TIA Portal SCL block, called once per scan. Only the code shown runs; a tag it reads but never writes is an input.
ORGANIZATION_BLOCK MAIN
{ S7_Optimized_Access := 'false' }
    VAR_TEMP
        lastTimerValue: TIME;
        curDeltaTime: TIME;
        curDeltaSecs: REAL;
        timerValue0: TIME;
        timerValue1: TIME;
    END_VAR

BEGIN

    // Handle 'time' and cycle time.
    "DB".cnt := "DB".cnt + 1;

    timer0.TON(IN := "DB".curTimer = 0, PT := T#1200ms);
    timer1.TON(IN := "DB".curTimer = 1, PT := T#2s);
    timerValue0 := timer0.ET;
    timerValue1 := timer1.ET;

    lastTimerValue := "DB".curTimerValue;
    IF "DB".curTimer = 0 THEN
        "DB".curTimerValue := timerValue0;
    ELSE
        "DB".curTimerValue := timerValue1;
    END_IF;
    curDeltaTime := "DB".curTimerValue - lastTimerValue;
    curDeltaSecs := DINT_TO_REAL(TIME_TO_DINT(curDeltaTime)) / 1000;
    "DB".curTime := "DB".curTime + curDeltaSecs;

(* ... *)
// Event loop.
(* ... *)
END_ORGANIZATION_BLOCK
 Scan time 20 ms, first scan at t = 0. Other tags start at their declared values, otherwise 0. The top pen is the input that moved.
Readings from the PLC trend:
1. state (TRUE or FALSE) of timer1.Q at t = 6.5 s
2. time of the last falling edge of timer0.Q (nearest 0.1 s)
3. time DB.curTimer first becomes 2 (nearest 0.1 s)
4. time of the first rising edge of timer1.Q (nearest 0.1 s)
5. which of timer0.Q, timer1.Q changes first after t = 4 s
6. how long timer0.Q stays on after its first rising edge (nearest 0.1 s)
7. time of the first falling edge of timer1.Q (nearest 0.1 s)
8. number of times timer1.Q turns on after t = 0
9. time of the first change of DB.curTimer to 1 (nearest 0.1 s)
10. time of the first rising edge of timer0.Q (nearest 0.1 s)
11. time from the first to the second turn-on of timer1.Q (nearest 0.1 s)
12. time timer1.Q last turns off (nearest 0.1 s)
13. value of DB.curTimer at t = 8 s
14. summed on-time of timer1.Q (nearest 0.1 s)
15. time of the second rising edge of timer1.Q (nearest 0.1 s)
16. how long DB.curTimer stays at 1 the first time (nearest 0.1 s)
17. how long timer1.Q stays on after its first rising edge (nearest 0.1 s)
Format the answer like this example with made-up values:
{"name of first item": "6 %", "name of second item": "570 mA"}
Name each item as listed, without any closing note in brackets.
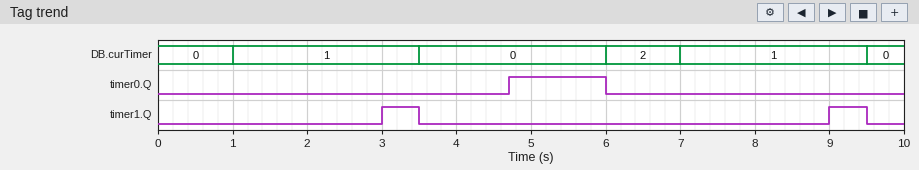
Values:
{"state (TRUE or FALSE) of timer1.Q at t = 6.5 s": "FALSE", "time of the last falling edge of timer0.Q": "6.0 s", "time DB.curTimer first becomes 2": "6.0 s", "time of the first rising edge of timer1.Q": "3.0 s", "which of timer0.Q, timer1.Q changes first after t = 4 s": "timer0.Q", "how long timer0.Q stays on after its first rising edge": "1.3 s", "time of the first falling edge of timer1.Q": "3.5 s", "number of times timer1.Q turns on after t = 0": "2", "time of the first change of DB.curTimer to 1": "1.0 s", "time of the first rising edge of timer0.Q": "4.7 s", "time from the first to the second turn-on of timer1.Q": "6.0 s", "time timer1.Q last turns off": "9.5 s", "value of DB.curTimer at t = 8 s": "1", "summed on-time of timer1.Q": "1.0 s", "time of the second rising edge of timer1.Q": "9.0 s", "how long DB.curTimer stays at 1 the first time": "2.5 s", "how long timer1.Q stays on after its first rising edge": "0.5 s"}
